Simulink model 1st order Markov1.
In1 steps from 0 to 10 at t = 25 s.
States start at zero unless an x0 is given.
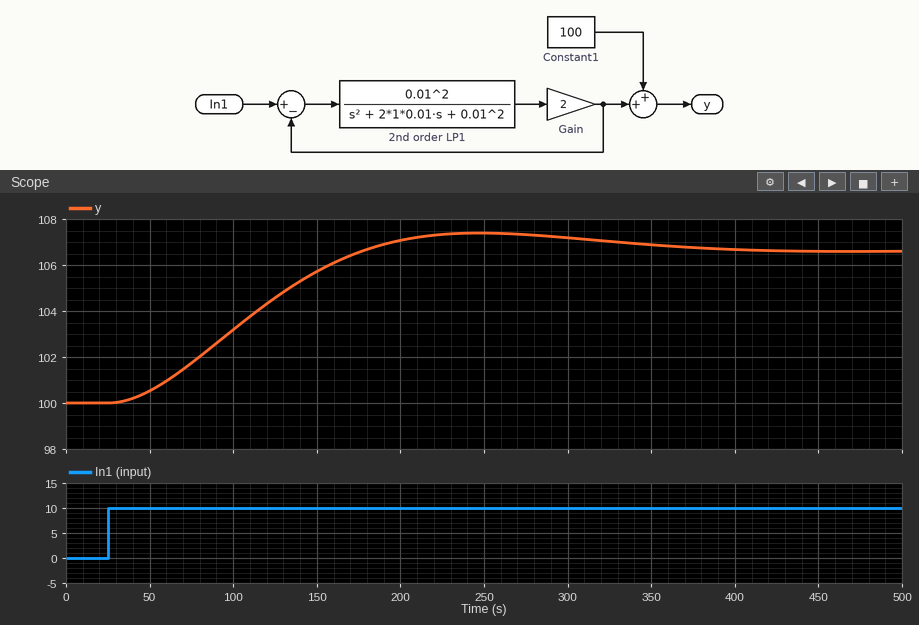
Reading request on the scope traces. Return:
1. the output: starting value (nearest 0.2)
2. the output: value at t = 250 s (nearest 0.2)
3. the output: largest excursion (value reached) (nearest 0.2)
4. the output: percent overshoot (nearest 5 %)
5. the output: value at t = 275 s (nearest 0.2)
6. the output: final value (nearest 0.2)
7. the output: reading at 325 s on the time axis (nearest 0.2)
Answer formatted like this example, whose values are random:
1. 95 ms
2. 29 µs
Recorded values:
1. 100.0
2. 107.4
3. 107.4
4. 10 %
5. 107.4
6. 106.6
7. 107.0
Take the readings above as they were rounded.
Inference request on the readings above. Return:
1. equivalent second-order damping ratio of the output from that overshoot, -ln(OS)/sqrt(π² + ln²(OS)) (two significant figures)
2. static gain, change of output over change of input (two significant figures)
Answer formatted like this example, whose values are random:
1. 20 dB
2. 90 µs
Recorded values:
1. 0.59
2. 0.66
